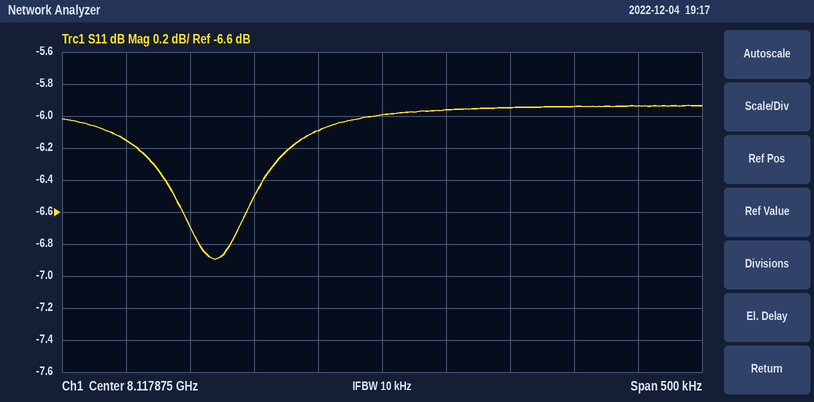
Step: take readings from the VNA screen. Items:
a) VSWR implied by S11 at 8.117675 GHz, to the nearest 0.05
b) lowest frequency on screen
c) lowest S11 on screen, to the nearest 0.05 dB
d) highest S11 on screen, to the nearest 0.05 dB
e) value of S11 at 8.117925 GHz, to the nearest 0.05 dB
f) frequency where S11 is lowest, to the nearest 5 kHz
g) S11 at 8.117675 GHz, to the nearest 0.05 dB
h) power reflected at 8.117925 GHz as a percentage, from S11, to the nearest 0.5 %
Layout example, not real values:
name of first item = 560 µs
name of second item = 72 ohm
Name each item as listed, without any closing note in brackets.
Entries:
VSWR implied by S11 at 8.117675 GHz, to the nearest 0.05 = 2.95
lowest frequency on screen = 8.117625 GHz
lowest S11 on screen, to the nearest 0.05 dB = -6.90 dB
highest S11 on screen, to the nearest 0.05 dB = -5.95 dB
value of S11 at 8.117925 GHz, to the nearest 0.05 dB = -5.95 dB
frequency where S11 is lowest, to the nearest 5 kHz = 8.117745 GHz
S11 at 8.117675 GHz, to the nearest 0.05 dB = -6.15 dB
power reflected at 8.117925 GHz as a percentage, from S11, to the nearest 0.5 % = 25.5 %
